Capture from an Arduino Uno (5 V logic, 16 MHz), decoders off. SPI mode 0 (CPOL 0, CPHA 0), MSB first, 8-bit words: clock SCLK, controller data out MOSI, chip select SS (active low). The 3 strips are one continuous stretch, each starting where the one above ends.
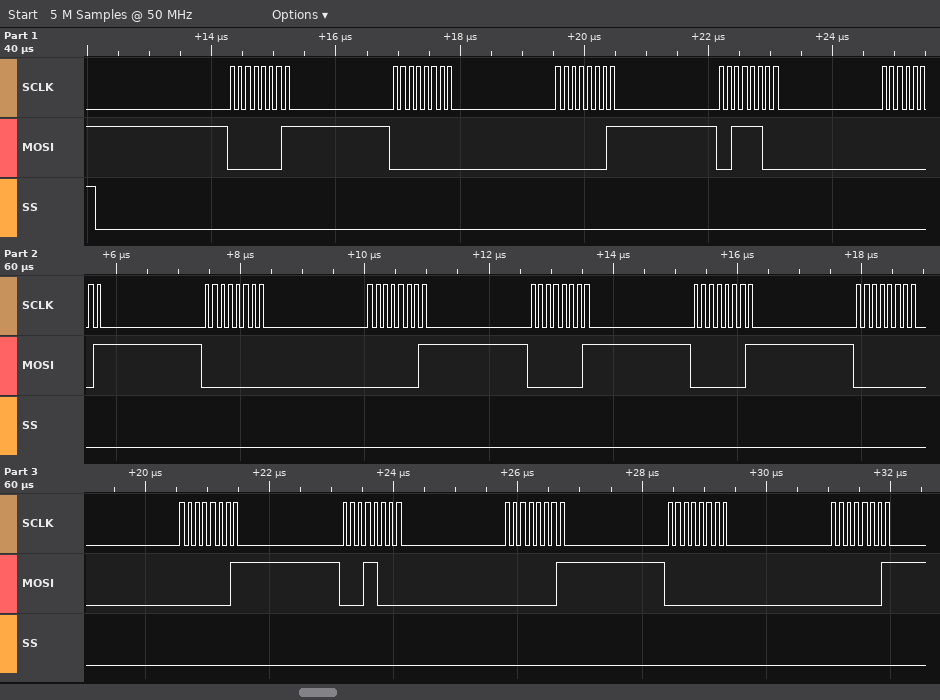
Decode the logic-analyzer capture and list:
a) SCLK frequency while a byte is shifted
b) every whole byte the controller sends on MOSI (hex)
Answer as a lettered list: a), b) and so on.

a) 8 MHz
b) 01 00 01 3C 01 00 01 01 01 00 01 18 01 00 01
